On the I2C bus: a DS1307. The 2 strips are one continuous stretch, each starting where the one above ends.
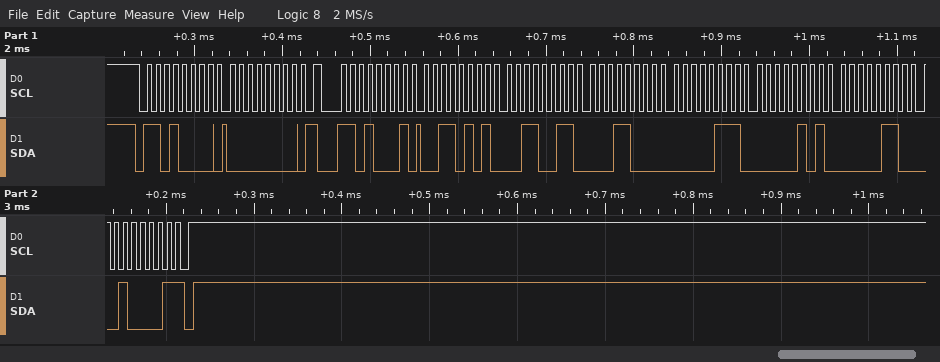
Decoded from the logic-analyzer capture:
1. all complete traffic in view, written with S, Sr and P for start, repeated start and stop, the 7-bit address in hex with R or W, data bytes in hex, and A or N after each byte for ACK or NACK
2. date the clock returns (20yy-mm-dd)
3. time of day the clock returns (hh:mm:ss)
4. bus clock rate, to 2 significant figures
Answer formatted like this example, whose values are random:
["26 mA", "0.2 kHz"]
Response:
["S 68W A 00 A Sr 68R A 35 A 33 A 18 A 07 A 05 A 06 A 21 N P", "2021-06-05", "18:33:35", "100 kHz"]
